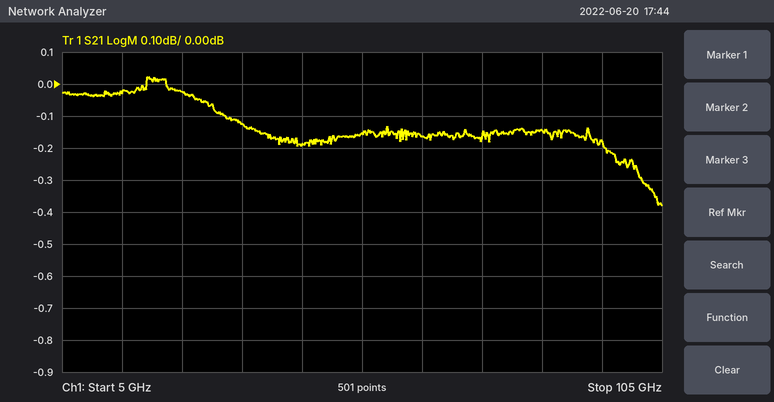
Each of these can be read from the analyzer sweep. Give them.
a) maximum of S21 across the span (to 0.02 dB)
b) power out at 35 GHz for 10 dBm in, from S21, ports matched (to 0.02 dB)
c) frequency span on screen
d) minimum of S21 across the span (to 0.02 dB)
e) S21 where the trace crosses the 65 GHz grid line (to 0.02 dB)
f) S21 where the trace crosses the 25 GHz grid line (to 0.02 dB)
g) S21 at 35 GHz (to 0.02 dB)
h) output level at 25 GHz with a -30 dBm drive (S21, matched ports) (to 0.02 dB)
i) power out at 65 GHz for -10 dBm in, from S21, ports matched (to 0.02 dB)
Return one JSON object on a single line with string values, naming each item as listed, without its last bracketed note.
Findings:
{"maximum of S21 across the span": "0.02 dB", "power out at 35 GHz for 10 dBm in, from S21, ports matched": "9.88 dBm", "frequency span on screen": "100 GHz", "minimum of S21 across the span": "-0.38 dB", "S21 where the trace crosses the 65 GHz grid line": "-0.16 dB", "S21 where the trace crosses the 25 GHz grid line": "-0.02 dB", "S21 at 35 GHz": "-0.12 dB", "output level at 25 GHz with a -30 dBm drive (S21, matched ports)": "-30.02 dBm", "power out at 65 GHz for -10 dBm in, from S21, ports matched": "-10.16 dBm"}
